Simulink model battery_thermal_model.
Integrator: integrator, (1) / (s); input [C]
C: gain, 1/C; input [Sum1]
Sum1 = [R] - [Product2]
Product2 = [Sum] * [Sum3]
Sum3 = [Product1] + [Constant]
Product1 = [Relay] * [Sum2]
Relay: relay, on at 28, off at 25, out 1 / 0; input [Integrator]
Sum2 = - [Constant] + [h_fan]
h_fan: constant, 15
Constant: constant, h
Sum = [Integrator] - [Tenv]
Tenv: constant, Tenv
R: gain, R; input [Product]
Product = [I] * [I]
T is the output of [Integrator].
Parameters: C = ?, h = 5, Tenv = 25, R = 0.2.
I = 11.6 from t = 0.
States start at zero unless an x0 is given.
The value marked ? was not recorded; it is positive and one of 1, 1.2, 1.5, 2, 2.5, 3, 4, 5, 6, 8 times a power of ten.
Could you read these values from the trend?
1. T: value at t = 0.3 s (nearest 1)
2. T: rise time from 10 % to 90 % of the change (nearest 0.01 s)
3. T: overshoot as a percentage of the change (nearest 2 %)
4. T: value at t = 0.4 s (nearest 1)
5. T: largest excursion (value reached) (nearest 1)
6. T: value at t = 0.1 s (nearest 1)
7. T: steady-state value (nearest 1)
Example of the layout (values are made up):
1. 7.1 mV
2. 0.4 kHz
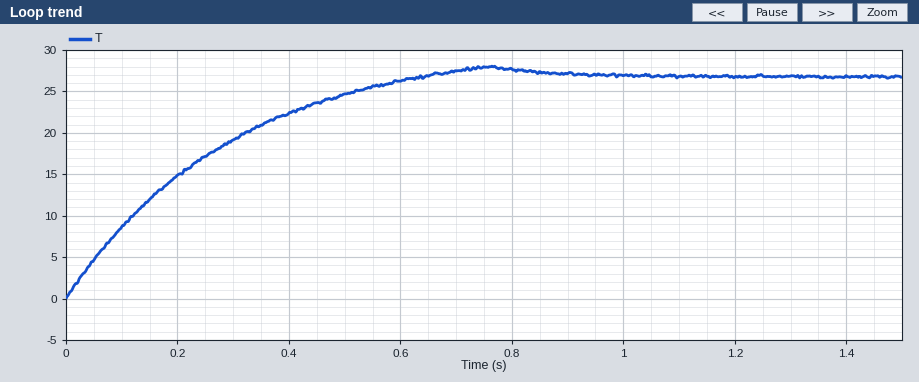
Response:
1. 19
2. 0.45 s
3. 4 %
4. 22
5. 28
6. 9
7. 27
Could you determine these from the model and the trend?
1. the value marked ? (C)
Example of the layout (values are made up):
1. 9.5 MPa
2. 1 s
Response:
1. 1.5
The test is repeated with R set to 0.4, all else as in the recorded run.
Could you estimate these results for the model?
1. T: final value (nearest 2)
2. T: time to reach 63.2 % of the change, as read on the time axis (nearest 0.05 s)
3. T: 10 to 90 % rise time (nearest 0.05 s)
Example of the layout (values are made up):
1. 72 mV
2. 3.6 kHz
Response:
1. 28
2. 0.20 s
3. 0.35 s
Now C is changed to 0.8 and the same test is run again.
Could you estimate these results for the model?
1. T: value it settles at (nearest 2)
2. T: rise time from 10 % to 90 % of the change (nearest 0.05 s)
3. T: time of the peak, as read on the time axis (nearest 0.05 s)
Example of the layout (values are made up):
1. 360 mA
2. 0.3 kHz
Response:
1. 26
2. 0.25 s
3. 0.40 s
